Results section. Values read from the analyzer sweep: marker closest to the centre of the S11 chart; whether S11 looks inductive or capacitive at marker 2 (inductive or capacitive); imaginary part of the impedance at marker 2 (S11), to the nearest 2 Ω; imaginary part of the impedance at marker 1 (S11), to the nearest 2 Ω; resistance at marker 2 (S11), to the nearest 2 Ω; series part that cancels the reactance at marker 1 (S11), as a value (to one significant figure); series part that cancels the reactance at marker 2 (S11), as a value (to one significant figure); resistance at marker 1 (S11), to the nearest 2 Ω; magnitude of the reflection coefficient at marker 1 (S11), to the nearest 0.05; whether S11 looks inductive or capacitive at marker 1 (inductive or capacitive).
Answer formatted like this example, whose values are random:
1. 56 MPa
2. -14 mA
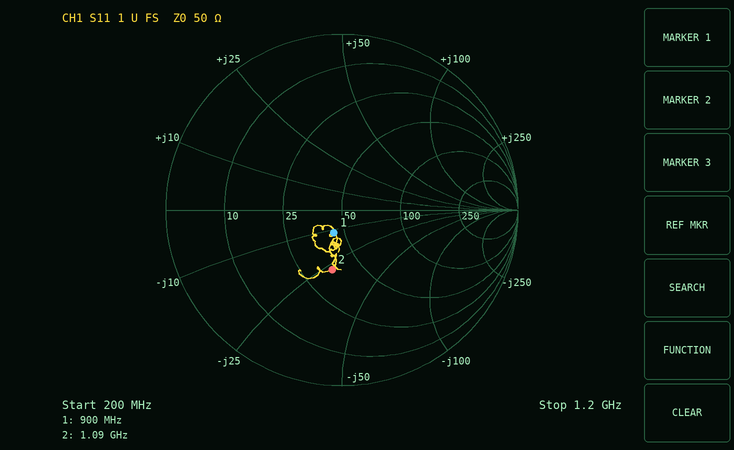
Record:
1. marker 1
2. capacitive
3. -28 Ω
4. -12 Ω
5. 36 Ω
6. 2 nH
7. 4 nH
8. 44 Ω
9. 0.15
10. capacitive
